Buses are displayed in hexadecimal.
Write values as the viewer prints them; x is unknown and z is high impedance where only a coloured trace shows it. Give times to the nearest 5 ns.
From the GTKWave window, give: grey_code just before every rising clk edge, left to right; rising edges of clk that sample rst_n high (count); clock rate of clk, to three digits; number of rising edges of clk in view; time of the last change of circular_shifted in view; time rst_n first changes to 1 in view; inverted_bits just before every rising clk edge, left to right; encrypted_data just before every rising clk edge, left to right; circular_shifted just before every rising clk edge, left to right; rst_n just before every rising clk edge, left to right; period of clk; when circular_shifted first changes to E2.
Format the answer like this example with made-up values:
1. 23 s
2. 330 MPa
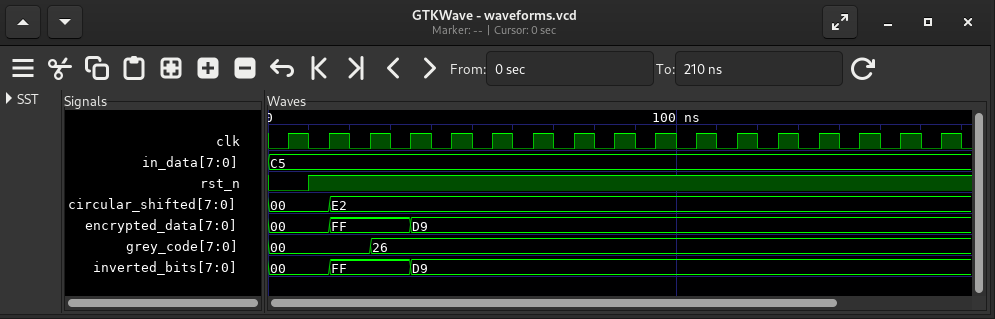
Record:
1. 00, 00, 00, 26, 26, 26, 26, 26, 26, 26, 26, 26, 26, 26, 26, 26, 26
2. 16
3. 100 MHz
4. 17
5. 15 ns
6. 10 ns
7. 00, 00, FF, FF, D9, D9, D9, D9, D9, D9, D9, D9, D9, D9, D9, D9, D9
8. 00, 00, FF, FF, D9, D9, D9, D9, D9, D9, D9, D9, D9, D9, D9, D9, D9
9. 00, 00, E2, E2, E2, E2, E2, E2, E2, E2, E2, E2, E2, E2, E2, E2, E2
10. 0 1 1 1 1 1 1 1 1 1 1 1 1 1 1 1 1
11. 10 ns
12. 15 ns
